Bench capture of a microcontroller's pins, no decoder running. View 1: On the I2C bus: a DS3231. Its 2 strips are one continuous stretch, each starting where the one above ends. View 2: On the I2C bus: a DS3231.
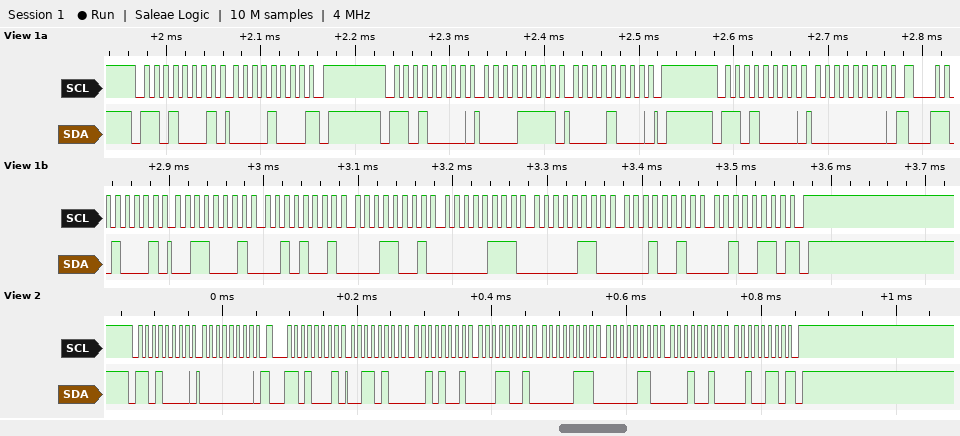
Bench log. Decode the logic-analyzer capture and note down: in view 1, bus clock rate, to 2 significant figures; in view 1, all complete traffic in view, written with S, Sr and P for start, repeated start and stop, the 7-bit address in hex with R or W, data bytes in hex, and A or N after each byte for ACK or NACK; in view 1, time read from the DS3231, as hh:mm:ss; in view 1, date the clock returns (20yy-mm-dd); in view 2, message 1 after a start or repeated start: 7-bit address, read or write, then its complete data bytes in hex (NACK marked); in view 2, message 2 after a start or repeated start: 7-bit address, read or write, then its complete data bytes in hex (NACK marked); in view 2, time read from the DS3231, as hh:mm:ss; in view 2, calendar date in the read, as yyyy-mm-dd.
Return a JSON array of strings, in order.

["100 kHz", "S 68R A 08 N P S 68W A 0F A 08 A P S 68W A 00 A Sr 68R A 31 A 29 A 19 A 07 A 06 A 12 A 26 N P", "19:29:31", "2026-12-06", "0x68 write: 00", "0x68 read: 34 29 19 07 06 12 26 NACK", "19:29:34", "2026-12-06"]
